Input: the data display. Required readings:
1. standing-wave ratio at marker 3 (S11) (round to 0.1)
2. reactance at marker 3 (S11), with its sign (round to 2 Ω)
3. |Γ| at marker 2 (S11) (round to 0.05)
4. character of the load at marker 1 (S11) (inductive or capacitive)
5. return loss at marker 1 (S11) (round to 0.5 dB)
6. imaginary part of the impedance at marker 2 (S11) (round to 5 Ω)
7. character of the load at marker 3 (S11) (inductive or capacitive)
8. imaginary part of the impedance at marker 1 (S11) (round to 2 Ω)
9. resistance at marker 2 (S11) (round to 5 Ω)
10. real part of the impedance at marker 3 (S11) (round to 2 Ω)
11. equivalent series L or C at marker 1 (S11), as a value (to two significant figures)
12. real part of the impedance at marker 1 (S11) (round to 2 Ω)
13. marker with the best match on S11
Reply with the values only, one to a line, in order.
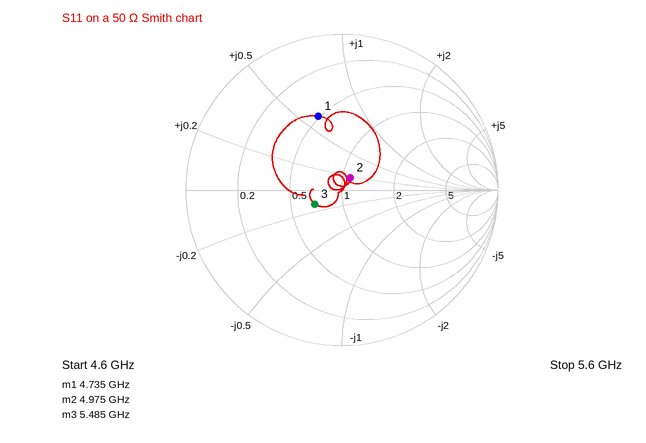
1.5
-6 Ω
0.10
inductive
6.0 dB
+10 Ω
capacitive
+30 Ω
55 Ω
34 Ω
1.0 nH
24 Ω
marker 2
